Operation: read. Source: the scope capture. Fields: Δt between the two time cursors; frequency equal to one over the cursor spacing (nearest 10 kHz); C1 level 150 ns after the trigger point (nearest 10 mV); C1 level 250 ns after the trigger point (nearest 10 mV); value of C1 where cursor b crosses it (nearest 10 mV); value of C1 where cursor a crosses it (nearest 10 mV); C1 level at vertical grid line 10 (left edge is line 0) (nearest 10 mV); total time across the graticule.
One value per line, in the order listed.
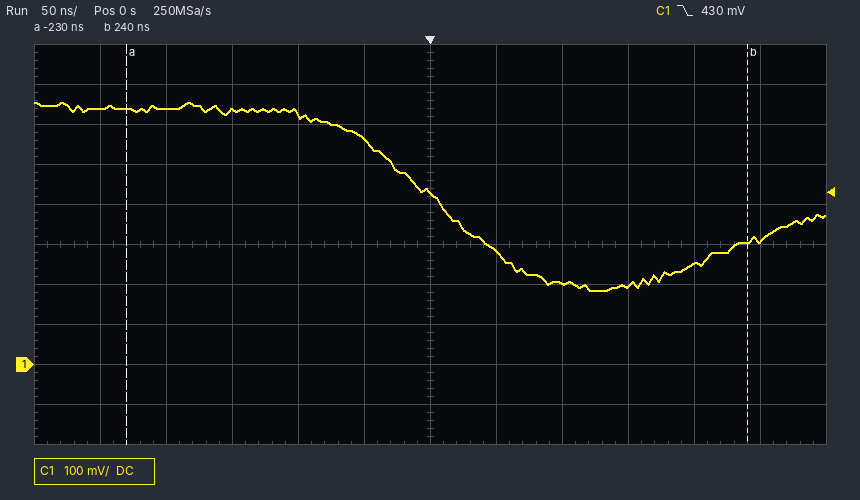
470 ns
2.13 MHz
200 mV
310 mV
310 mV
640 mV
250 mV
600 ns
